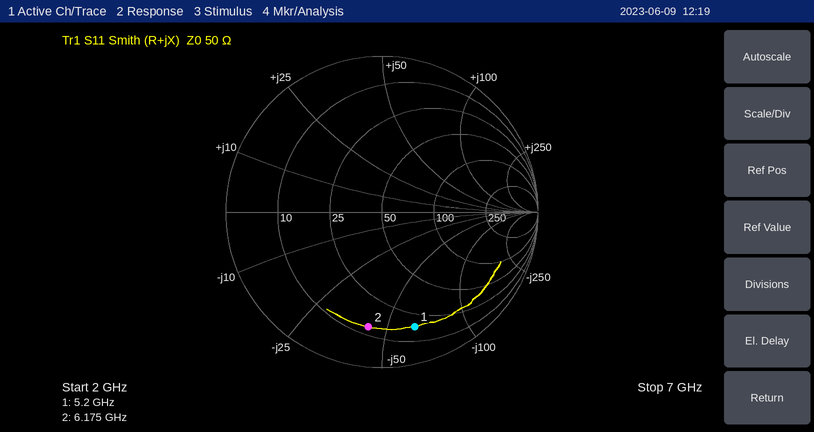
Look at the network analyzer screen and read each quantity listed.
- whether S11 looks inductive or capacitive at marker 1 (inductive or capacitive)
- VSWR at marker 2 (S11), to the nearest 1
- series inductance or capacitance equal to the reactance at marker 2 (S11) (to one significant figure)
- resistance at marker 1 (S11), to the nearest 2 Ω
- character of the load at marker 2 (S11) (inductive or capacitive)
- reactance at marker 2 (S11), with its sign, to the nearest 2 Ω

capacitive
7
600 fF
18 Ω
capacitive
-42 Ω
